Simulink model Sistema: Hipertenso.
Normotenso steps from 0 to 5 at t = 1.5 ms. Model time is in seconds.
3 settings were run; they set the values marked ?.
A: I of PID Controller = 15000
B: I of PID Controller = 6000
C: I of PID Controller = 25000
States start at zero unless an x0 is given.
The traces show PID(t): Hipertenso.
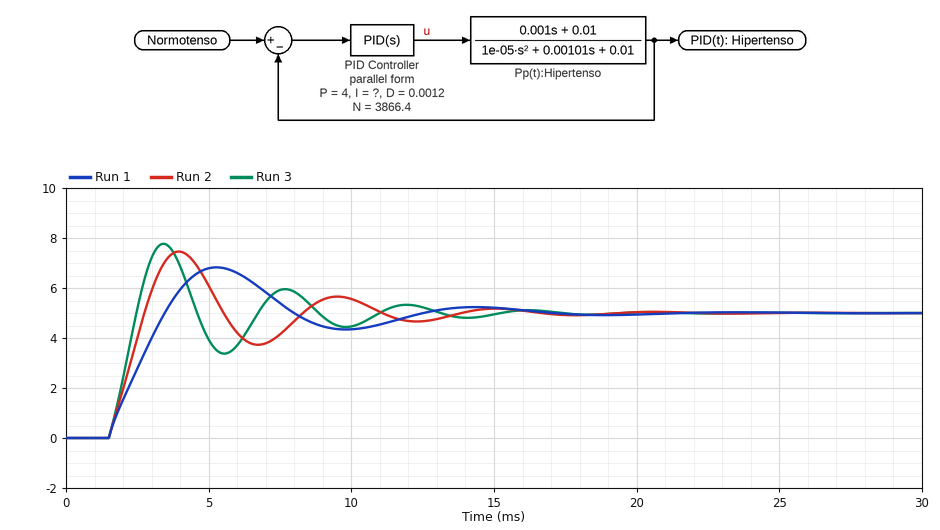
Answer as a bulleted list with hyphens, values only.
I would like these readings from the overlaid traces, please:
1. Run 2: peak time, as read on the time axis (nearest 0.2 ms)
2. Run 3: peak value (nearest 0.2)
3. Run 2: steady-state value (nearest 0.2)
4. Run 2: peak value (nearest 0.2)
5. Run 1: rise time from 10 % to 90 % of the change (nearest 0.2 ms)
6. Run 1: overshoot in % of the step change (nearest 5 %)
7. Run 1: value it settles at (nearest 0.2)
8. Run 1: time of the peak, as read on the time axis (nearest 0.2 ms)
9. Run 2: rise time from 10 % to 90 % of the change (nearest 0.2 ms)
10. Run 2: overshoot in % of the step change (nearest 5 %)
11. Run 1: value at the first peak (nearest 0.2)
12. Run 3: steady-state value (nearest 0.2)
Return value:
- 4.0 ms
- 7.8
- 5.0
- 7.4
- 1.6 ms
- 35 %
- 5.0
- 5.2 ms
- 1.0 ms
- 50 %
- 6.8
- 5.0
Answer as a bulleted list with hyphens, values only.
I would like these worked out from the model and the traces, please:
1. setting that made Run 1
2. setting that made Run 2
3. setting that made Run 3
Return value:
- B
- A
- C
